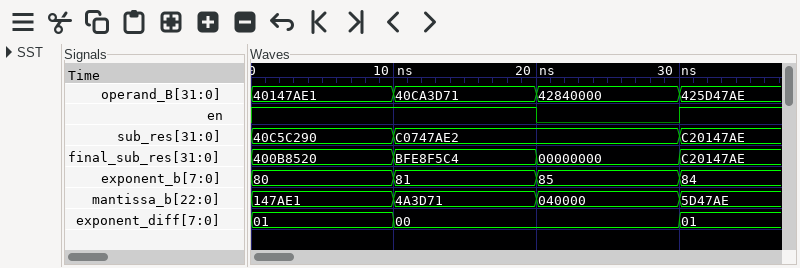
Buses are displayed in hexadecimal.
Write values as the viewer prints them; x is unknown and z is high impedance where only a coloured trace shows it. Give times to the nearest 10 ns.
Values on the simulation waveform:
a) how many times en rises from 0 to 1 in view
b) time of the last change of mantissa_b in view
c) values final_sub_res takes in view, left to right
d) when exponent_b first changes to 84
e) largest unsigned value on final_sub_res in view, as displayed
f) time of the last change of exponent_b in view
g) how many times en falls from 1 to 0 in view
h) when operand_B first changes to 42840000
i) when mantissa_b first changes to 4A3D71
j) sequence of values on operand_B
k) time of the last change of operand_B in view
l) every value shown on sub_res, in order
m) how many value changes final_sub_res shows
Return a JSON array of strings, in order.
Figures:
["1", "30 ns", "400B8520, BFE8F5C4, 00000000, C20147AE", "30 ns", "C20147AE", "30 ns", "1", "20 ns", "10 ns", "40147AE1, 40CA3D71, 42840000, 425D47AE", "30 ns", "40C5C290, C0747AE2, C20147AE", "3"]
